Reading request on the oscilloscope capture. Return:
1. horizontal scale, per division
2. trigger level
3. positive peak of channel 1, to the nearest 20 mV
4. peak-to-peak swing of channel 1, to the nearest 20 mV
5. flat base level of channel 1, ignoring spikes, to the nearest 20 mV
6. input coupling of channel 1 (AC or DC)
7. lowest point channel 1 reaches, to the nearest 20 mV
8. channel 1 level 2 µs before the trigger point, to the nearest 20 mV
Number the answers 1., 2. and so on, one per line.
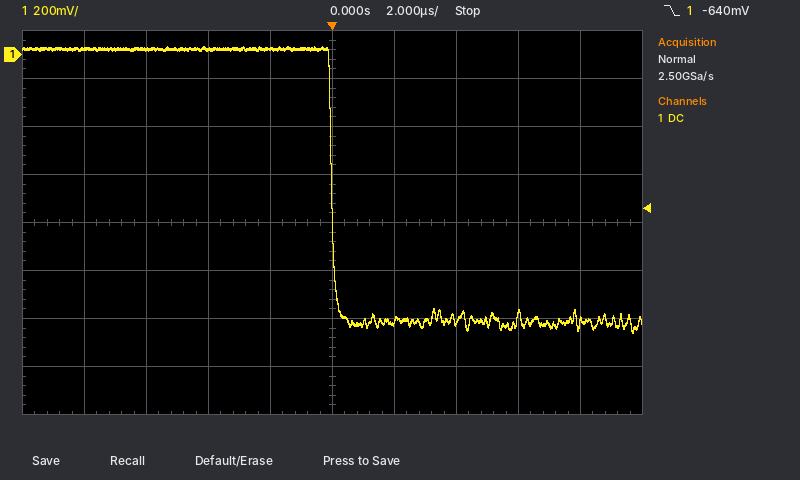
1. 2 µs
2. -640 mV
3. 40 mV
4. 1.20 V
5. -1.12 V
6. DC
7. -1.16 V
8. 20 mV
